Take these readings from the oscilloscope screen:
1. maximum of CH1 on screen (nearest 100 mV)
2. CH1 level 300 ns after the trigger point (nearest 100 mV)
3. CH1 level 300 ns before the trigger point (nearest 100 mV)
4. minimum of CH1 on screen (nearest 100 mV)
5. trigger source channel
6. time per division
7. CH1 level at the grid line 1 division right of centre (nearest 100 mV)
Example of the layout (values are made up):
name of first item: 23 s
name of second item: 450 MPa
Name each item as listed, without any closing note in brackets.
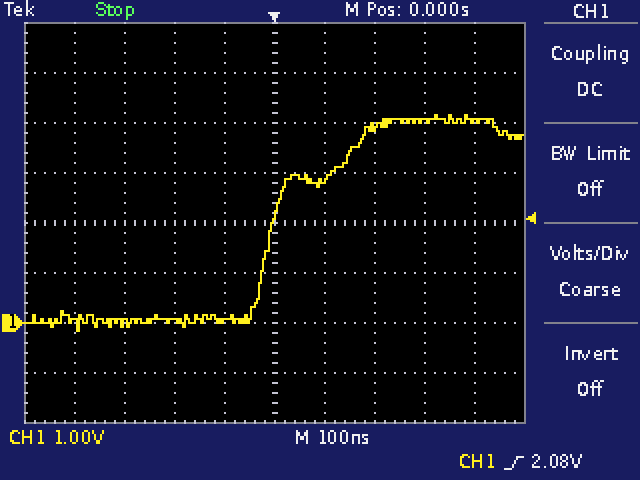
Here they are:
maximum of CH1 on screen: 4.2 V
CH1 level 300 ns after the trigger point: 4.0 V
CH1 level 300 ns before the trigger point: 0.0 V
minimum of CH1 on screen: -200 mV
trigger source channel: CH1
time per division: 100 ns
CH1 level at the grid line 1 division right of centre: 2.9 V
